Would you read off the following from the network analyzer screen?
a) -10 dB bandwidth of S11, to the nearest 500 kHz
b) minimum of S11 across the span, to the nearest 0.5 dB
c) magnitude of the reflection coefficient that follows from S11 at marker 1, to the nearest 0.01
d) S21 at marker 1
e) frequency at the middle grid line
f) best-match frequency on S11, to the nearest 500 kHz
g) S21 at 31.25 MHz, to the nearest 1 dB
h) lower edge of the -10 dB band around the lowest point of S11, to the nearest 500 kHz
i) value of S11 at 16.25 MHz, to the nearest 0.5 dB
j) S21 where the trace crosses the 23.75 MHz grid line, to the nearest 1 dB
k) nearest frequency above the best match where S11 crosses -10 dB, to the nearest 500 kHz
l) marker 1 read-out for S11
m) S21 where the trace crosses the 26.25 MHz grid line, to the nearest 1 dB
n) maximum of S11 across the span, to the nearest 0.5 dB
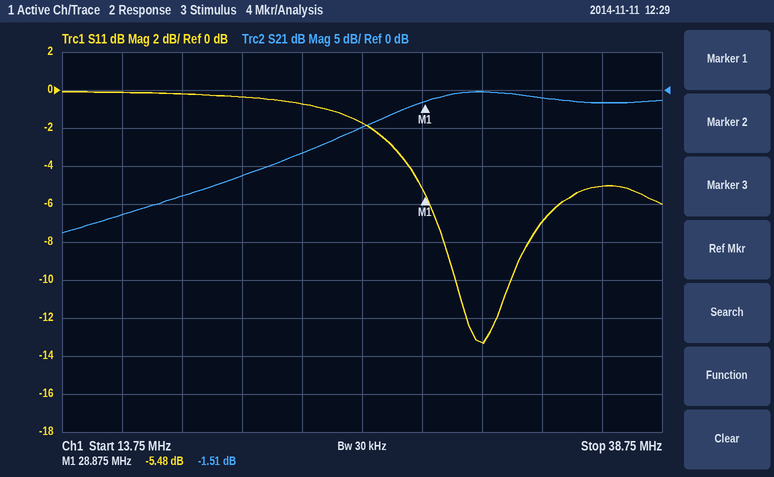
2.5 MHz
-13.5 dB
0.53
-1.51 dB
26.25 MHz
31.5 MHz
0 dB
30.0 MHz
0.0 dB
-8 dB
32.5 MHz
-5.48 dB
-5 dB
0.0 dB
